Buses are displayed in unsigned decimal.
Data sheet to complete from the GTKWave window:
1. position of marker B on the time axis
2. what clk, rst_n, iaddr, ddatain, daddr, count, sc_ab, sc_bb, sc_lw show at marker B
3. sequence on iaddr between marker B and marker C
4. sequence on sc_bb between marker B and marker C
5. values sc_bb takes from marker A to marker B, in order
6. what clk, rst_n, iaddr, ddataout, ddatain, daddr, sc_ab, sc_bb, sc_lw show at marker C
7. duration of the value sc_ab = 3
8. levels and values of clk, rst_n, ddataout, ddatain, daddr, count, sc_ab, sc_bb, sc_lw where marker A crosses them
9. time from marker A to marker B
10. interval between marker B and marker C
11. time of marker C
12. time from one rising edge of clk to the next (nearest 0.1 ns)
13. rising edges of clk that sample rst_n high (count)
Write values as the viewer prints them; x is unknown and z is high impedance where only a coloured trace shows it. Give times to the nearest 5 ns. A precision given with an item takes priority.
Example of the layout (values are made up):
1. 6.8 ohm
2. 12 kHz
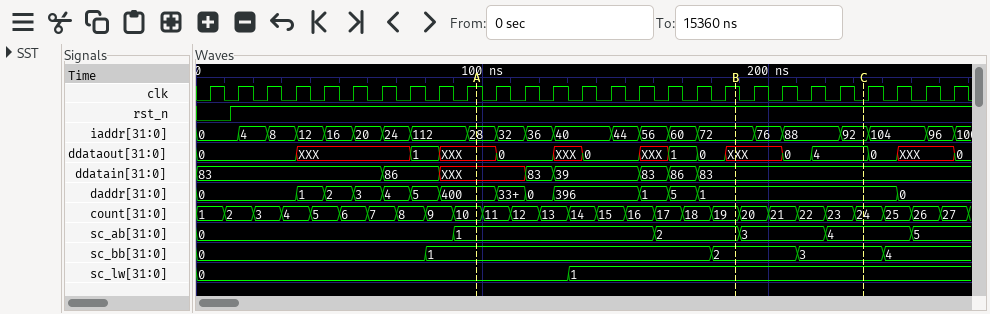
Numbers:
1. 190 ns
2. clk=1, rst_n=1, iaddr=72, ddatain=83, daddr=1, count=19, sc_ab=2, sc_bb=2, sc_lw=1
3. 72, 76, 88, 92
4. 2, 3
5. 1, 2
6. clk=0, rst_n=1, iaddr=92, ddataout=4, ddatain=83, daddr=1, sc_ab=4, sc_bb=3, sc_lw=1
7. 30 ns
8. clk=1, rst_n=1, ddataout=XXX, ddatain=XXX, daddr=400, count=10, sc_ab=1, sc_bb=1, sc_lw=0
9. 90 ns
10. 45 ns
11. 235 ns
12. 10 ns
13. 26
